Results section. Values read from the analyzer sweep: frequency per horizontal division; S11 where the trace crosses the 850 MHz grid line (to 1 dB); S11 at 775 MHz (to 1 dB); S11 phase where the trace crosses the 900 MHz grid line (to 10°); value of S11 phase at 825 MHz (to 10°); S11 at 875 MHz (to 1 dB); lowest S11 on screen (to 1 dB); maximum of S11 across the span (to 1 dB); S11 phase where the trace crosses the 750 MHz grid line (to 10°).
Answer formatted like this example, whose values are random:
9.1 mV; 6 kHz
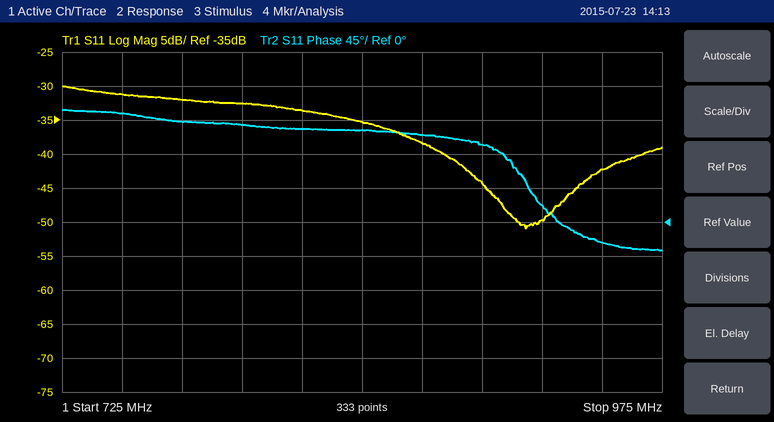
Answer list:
25 MHz; -35 dB; -32 dB; 100°; 120°; -38 dB; -51 dB; -30 dB; 140°
